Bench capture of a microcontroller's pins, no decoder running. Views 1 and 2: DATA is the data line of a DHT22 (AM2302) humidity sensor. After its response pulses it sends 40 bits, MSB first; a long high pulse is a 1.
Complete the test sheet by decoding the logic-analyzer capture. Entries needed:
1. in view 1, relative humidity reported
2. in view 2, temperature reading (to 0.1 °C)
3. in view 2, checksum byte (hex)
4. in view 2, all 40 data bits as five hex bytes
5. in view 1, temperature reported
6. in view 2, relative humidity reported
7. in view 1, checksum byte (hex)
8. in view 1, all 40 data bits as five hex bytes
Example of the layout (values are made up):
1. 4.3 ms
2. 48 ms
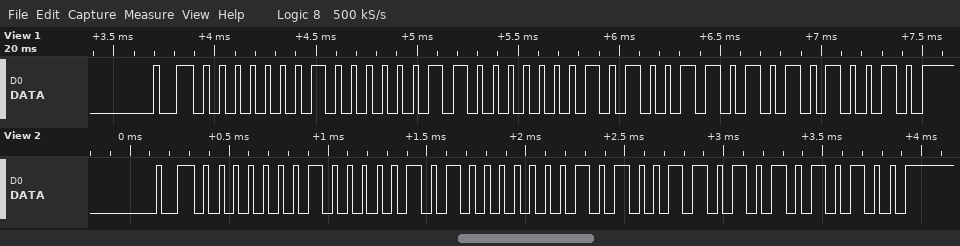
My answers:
1. 25.9 %
2. 33.3 °C
3. 0x54
4. 01 05 01 4D 54
5. 33.3 °C
6. 26.1 %
7. 0x52
8. 01 03 01 4D 52
